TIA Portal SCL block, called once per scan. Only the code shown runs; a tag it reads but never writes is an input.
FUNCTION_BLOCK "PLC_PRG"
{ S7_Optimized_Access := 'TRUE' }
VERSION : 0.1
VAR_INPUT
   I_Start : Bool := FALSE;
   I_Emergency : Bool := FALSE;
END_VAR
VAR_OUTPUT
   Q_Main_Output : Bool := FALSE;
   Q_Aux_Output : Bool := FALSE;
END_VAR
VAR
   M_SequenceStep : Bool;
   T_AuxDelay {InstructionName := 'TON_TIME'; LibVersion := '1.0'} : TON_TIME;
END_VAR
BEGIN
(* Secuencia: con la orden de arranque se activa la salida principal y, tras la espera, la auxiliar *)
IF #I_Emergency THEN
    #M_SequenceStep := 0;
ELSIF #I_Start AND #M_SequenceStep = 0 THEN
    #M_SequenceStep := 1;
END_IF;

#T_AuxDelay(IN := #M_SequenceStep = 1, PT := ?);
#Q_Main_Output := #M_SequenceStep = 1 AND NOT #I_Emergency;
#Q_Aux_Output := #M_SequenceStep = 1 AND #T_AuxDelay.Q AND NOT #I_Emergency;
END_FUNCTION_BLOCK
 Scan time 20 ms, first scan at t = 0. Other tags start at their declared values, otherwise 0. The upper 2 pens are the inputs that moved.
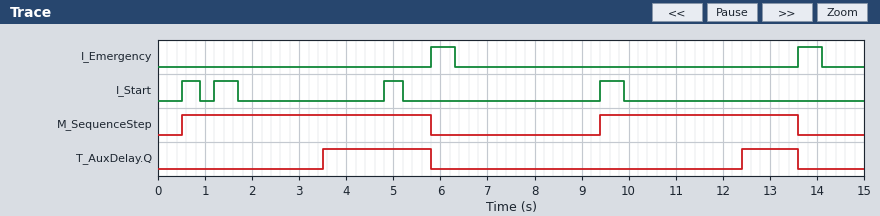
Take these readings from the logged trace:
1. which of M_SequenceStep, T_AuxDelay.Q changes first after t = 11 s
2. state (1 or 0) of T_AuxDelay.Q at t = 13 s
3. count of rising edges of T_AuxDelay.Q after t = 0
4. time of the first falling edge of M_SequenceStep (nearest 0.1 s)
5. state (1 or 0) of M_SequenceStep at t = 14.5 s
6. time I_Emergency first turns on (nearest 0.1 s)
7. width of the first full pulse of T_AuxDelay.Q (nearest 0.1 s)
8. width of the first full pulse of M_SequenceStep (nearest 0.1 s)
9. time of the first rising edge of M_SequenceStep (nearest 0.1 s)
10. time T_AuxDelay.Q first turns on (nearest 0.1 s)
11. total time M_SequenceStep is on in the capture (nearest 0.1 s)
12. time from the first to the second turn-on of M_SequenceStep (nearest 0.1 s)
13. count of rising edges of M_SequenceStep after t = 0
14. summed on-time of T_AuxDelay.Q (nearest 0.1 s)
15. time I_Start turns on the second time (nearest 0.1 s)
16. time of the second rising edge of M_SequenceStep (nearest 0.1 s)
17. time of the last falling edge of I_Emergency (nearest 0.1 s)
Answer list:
T_AuxDelay.Q
1
2
5.8 s
0
5.8 s
2.3 s
5.3 s
0.5 s
3.5 s
9.5 s
8.9 s
2
3.5 s
1.2 s
9.4 s
14.1 s
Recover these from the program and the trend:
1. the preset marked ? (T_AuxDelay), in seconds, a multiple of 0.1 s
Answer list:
3.0 s
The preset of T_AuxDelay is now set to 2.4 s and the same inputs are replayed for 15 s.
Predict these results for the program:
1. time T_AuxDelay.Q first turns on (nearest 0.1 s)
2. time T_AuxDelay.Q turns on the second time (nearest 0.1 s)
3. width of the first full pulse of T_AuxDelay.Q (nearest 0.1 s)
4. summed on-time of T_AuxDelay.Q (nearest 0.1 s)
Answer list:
2.9 s
11.8 s
2.9 s
4.7 s
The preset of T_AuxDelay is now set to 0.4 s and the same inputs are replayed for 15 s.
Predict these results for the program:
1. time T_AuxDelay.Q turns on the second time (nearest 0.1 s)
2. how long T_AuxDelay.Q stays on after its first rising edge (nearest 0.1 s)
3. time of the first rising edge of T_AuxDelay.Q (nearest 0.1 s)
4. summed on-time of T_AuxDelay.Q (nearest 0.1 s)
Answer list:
9.8 s
4.9 s
0.9 s
8.7 s
